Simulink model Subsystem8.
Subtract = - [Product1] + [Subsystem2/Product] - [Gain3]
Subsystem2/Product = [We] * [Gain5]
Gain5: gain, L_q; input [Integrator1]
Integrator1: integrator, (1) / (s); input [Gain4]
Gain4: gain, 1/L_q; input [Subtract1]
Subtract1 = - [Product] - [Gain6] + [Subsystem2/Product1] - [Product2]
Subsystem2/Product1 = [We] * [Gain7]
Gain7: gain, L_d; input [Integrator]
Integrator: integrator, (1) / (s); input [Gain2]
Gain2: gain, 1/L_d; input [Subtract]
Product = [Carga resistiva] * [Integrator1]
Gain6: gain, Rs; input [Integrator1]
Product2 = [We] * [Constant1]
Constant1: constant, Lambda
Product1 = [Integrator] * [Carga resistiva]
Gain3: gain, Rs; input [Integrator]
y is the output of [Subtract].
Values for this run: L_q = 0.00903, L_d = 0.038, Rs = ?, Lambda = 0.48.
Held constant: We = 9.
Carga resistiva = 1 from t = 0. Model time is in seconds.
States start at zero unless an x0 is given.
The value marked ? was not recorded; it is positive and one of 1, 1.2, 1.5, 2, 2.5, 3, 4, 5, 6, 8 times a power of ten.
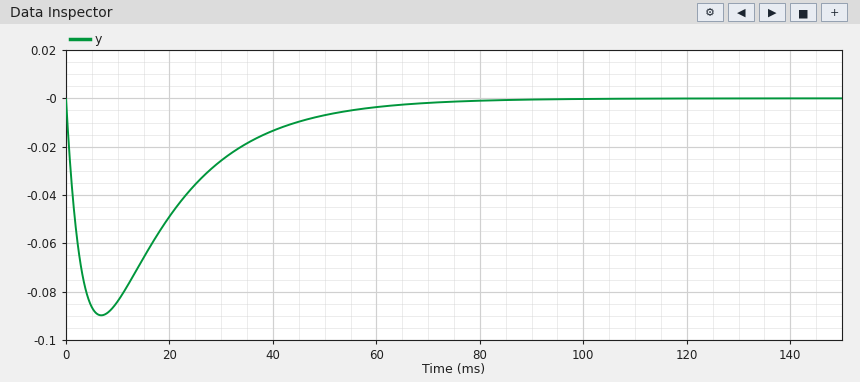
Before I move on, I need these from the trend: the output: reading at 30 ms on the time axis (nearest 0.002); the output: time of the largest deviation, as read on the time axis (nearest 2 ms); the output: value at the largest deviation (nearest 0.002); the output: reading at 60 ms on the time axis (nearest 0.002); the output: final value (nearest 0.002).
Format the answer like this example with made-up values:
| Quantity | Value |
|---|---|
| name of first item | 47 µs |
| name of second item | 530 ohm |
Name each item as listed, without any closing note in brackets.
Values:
| Quantity | Value |
|---|---|
| the output: reading at 30 ms on the time axis | -0.026 |
| the output: time of the largest deviation, as read on the time axis | 6 ms |
| the output: value at the largest deviation | -0.090 |
| the output: reading at 60 ms on the time axis | -0.004 |
| the output: final value | 0.000 |
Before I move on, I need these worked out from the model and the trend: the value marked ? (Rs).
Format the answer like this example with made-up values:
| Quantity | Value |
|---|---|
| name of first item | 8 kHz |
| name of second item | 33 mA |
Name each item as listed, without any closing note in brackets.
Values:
| Quantity | Value |
|---|---|
| the value marked ? | 1.5 |
